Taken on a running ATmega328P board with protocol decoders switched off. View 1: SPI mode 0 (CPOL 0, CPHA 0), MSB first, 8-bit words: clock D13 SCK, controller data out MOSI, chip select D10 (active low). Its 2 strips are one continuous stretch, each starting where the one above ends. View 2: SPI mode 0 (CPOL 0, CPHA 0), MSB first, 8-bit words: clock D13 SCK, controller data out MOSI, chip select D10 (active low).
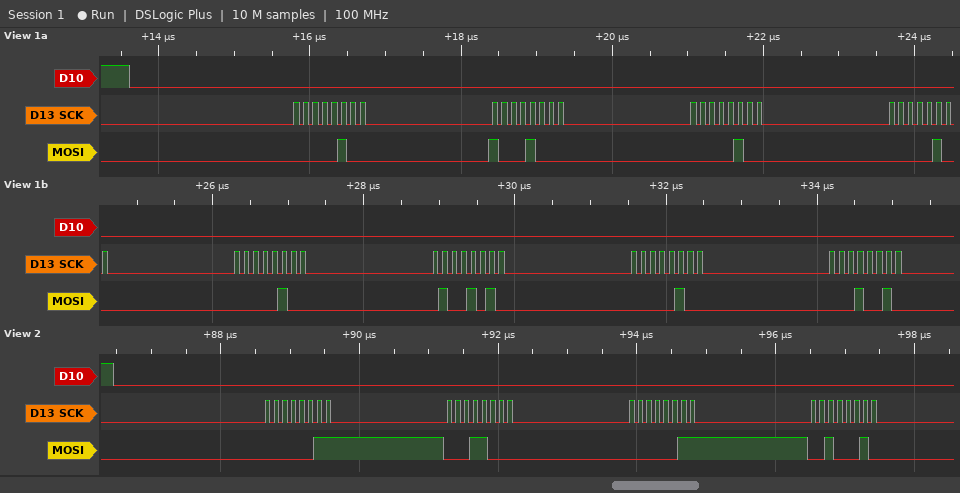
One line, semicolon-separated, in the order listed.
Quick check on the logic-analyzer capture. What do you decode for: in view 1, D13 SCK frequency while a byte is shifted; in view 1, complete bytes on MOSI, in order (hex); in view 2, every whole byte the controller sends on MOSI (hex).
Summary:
8 MHz; 0x04 0x88 0x04 0x04 0x04 0x4A 0x04 0x12; 0x03 0x18 0x03 0x22
